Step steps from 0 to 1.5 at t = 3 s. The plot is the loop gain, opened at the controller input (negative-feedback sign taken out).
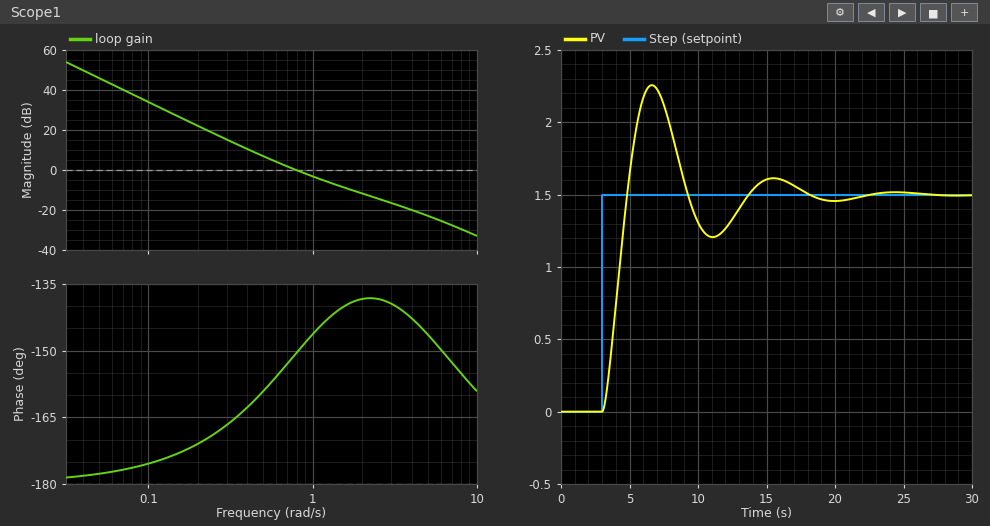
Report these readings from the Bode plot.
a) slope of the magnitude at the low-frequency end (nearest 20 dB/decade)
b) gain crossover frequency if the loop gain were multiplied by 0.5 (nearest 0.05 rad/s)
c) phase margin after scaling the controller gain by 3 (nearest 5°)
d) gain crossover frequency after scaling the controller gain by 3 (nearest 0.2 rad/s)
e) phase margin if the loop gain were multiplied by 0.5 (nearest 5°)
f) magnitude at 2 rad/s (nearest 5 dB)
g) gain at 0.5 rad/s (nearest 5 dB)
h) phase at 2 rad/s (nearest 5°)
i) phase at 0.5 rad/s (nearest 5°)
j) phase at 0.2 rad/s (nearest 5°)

-40 dB/decade
0.55 rad/s
40°
1.6 rad/s
20°
-10 dB
5 dB
-140°
-160°
-170°
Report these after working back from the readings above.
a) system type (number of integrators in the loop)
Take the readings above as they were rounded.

2
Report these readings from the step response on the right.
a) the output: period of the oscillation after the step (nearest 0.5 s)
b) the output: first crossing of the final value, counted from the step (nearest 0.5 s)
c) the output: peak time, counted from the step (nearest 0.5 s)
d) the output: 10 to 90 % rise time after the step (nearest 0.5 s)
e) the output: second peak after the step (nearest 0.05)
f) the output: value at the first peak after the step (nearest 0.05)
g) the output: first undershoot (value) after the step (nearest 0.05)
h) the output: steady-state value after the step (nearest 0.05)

9.0 s
2.0 s
3.5 s
1.5 s
1.60
2.25
1.20
1.50
